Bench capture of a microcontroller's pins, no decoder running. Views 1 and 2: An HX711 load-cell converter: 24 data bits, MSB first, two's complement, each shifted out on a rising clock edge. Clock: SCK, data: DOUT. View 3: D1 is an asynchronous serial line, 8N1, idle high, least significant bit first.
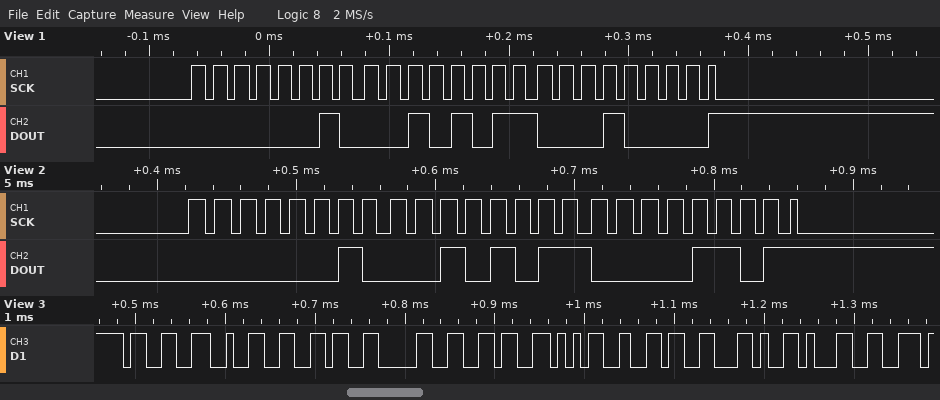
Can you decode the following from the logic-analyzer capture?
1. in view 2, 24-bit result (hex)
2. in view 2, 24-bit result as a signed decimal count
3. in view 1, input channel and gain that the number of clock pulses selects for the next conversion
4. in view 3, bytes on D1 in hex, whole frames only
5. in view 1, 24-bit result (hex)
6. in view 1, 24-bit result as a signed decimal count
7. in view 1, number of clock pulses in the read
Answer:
0x022B0D
142093
channel A, gain 128
33 32 36 30 36 35 36 2C 31
0x022B10
142096
25
